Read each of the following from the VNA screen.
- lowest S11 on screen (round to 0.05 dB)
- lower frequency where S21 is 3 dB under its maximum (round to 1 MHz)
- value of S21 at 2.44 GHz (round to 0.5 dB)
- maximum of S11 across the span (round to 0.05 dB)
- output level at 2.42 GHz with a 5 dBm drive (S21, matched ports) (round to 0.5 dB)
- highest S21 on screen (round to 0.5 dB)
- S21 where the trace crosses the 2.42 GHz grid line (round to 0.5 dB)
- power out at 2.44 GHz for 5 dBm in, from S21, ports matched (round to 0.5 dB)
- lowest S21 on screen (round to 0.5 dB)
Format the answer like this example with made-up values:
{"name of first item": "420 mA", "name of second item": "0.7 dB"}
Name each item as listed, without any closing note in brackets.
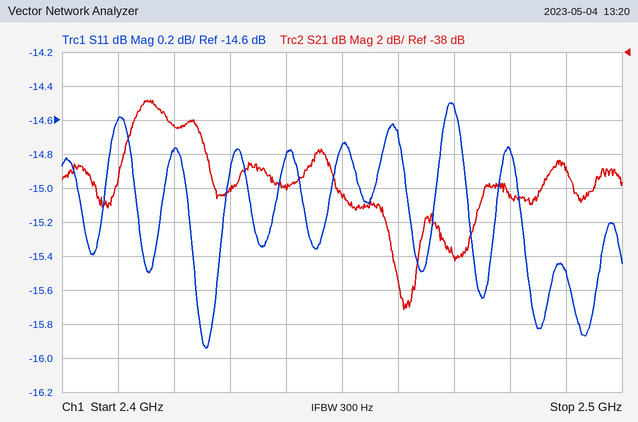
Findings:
{"lowest S11 on screen": "-15.95 dB", "lower frequency where S21 is 3 dB under its maximum": "2.411 GHz", "value of S21 at 2.44 GHz": "-46.0 dB", "maximum of S11 across the span": "-14.50 dB", "output level at 2.42 GHz with a 5 dBm drive (S21, matched ports)": "-37.5 dBm", "highest S21 on screen": "-41.0 dB", "S21 where the trace crosses the 2.42 GHz grid line": "-42.5 dB", "power out at 2.44 GHz for 5 dBm in, from S21, ports matched": "-41.0 dBm", "lowest S21 on screen": "-53.0 dB"}
